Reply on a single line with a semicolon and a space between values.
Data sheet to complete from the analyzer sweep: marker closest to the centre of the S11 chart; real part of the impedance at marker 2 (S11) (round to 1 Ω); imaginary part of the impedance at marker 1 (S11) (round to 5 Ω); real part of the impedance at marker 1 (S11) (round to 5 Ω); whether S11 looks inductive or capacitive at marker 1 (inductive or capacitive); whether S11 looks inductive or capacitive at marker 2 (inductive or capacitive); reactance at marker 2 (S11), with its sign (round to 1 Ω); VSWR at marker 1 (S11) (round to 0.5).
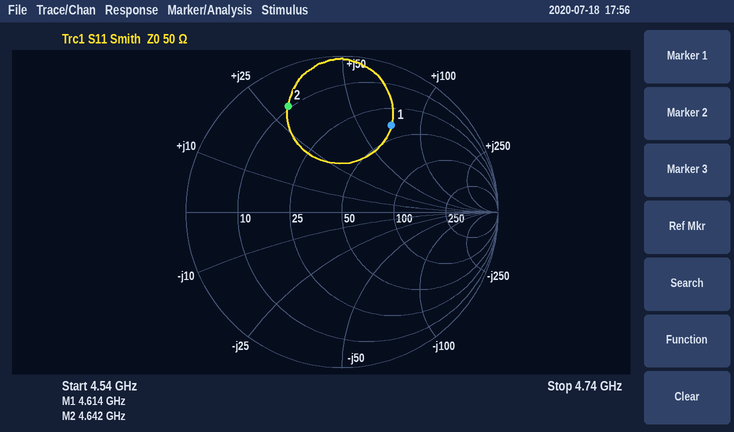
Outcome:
marker 1; 9 Ω; +70 Ω; 40 Ω; inductive; inductive; +30 Ω; 4.5
